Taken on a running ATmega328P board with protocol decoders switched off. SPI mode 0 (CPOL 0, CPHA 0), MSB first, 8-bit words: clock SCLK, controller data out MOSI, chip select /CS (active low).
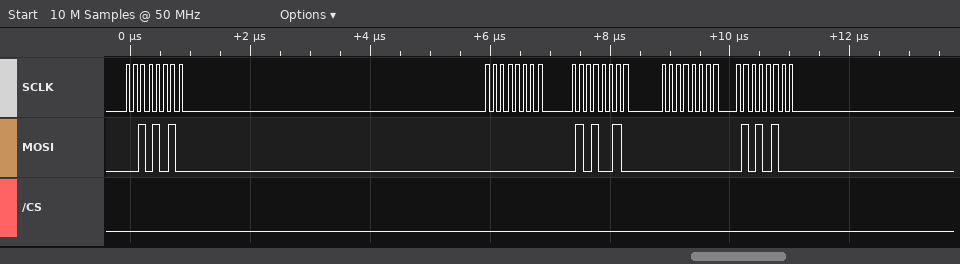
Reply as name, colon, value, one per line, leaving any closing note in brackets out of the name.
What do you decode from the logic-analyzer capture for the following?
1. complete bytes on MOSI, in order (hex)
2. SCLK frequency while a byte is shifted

complete bytes on MOSI, in order: 2A 00 52 00 54
SCLK frequency while a byte is shifted: 8 MHz
